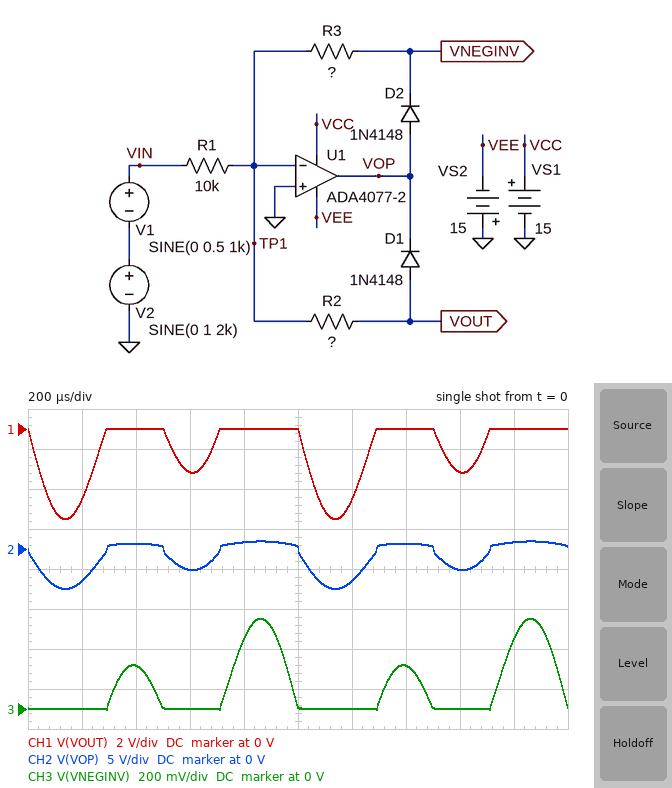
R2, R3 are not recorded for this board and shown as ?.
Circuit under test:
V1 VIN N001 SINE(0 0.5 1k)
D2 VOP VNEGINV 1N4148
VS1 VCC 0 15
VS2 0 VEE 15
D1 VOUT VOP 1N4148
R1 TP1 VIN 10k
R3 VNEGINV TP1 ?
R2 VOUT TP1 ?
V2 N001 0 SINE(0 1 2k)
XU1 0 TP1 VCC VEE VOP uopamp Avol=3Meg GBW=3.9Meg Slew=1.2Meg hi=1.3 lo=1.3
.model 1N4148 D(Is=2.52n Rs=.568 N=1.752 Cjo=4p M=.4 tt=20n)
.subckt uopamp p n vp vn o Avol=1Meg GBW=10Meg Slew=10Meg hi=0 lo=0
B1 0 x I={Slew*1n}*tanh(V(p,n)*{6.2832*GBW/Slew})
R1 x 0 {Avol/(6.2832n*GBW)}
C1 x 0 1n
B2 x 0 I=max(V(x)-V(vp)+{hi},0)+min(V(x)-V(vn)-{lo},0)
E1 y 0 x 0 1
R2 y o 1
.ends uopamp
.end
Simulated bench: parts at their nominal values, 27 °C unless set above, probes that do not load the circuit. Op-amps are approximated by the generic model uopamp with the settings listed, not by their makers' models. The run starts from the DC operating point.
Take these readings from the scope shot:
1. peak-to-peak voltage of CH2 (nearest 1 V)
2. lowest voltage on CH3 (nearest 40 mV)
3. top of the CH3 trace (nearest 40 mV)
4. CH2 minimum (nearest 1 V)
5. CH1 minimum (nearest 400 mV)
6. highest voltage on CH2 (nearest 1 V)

6 V
0 V
440 mV
-5 V
-4.4 V
1 V
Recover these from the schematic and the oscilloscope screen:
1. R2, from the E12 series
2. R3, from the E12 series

33 kΩ
3.3 kΩ
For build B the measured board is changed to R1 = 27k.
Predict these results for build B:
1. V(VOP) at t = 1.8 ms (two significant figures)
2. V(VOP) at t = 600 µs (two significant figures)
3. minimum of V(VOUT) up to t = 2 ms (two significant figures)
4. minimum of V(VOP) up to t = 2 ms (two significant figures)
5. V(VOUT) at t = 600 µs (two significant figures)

570 mV
-1.2 V
-1.7 V
-2.1 V
-800 mV
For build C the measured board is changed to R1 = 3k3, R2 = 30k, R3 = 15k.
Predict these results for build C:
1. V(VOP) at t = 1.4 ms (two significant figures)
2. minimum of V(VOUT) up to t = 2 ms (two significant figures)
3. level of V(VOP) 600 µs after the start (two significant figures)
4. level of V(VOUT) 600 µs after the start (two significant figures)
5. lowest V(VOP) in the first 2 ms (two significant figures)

3.5 V
-12 V
-6.5 V
-6.0 V
-13 V
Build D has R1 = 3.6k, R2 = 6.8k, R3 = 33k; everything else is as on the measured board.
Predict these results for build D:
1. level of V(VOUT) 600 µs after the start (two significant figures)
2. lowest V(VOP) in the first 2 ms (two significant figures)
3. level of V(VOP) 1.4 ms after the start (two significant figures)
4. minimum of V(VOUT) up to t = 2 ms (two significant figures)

-1.2 V
-3.1 V
6.5 V
-2.6 V
